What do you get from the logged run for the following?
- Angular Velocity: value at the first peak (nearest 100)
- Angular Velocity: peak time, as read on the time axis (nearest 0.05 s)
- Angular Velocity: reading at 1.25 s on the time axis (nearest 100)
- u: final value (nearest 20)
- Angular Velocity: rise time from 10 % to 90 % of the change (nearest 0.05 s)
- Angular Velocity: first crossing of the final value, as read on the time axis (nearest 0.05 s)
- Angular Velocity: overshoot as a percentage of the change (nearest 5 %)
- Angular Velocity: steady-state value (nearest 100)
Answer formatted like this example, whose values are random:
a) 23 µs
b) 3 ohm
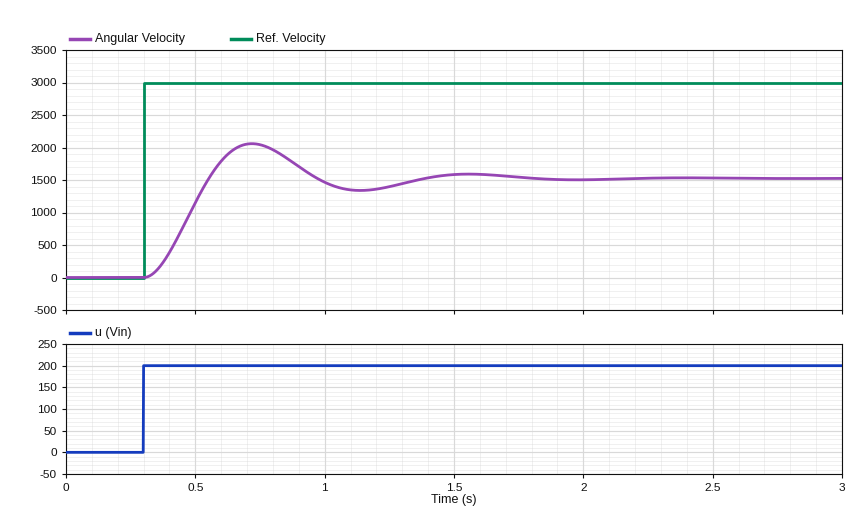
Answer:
a) 2100
b) 0.70 s
c) 1400
d) 200
e) 0.15 s
f) 0.55 s
g) 35 %
h) 1500
